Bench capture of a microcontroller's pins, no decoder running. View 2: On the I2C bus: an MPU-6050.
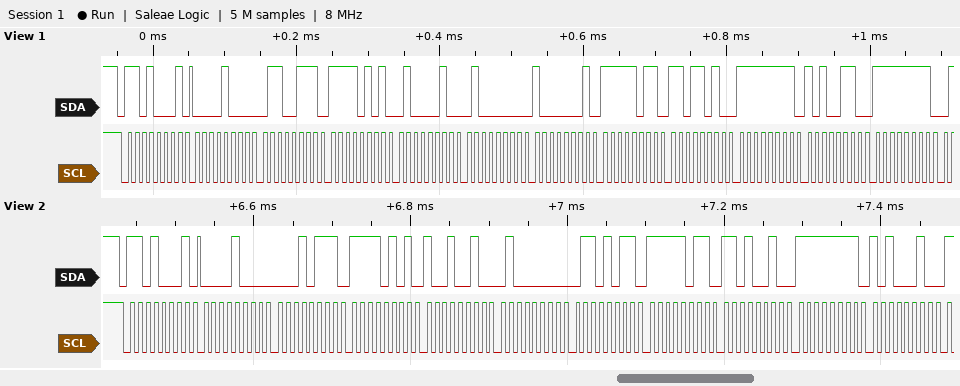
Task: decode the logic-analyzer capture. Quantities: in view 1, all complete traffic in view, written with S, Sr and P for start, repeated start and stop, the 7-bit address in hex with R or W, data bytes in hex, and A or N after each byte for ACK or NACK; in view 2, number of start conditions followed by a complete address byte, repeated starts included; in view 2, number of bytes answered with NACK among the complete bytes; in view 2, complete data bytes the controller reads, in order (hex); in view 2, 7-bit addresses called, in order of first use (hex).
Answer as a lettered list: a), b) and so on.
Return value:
a) S 68R A 08 A 67 A F5 A 42 A 40 A 81 A FB A DA A FF A A6 A FF A
b) 1
c) 0
d) 08 17 F5 92 40 6B FB D2 FF A2
e) 0x68
